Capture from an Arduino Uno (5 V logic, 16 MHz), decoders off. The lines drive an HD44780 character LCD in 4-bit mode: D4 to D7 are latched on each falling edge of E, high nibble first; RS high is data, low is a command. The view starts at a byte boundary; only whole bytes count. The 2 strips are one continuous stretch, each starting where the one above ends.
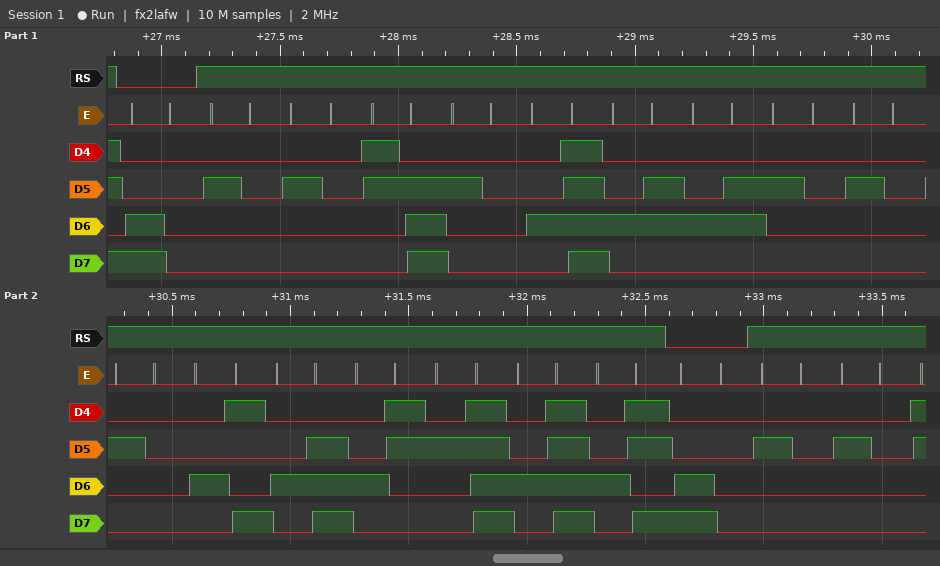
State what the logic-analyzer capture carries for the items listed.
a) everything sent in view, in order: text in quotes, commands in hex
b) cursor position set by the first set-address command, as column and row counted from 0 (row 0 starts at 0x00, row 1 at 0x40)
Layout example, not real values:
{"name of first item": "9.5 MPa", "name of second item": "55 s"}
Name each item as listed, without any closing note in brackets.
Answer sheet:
{"everything sent in view, in order: text in quotes, commands in hex": "0xC0 \"  > OFF   INC/OK\" 0xC0 \"  \"", "cursor position set by the first set-address command, as column and row counted from 0": "column 0, row 1"}
